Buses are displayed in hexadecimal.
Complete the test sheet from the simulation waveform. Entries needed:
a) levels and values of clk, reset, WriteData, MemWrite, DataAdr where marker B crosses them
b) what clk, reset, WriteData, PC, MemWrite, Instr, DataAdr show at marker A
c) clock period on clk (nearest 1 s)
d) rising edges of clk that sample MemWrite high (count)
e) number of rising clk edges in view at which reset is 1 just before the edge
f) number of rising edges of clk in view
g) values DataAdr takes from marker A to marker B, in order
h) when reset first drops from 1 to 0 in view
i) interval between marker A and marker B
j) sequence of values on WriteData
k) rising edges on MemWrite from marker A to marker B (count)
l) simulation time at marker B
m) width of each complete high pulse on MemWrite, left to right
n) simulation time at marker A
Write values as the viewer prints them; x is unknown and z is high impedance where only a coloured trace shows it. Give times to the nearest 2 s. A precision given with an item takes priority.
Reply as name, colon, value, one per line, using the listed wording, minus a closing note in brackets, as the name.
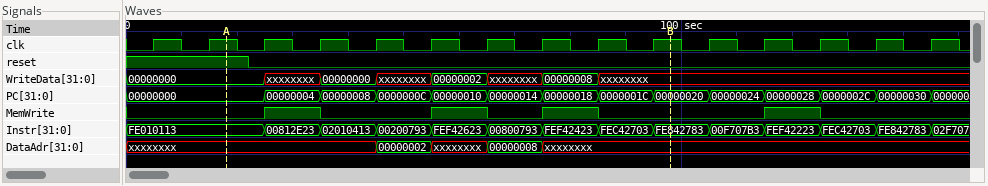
levels and values of clk, reset, WriteData, MemWrite, DataAdr where marker B crosses them: clk=1, reset=0, WriteData=xxxxxxxx, MemWrite=0, DataAdr=xxxxxxxx
what clk, reset, WriteData, PC, MemWrite, Instr, DataAdr show at marker A: clk=1, reset=1, WriteData=00000000, PC=00000000, MemWrite=0, Instr=FE010113, DataAdr=xxxxxxxx
clock period on clk: 10 s
rising edges of clk that sample MemWrite high: 4
number of rising clk edges in view at which reset is 1 just before the edge: 2
number of rising edges of clk in view: 15
values DataAdr takes from marker A to marker B, in order: xxxxxxxx, 00000002, xxxxxxxx, 00000008, xxxxxxxx
when reset first drops from 1 to 0 in view: 22 s
interval between marker A and marker B: 80 s
sequence of values on WriteData: 00000000, xxxxxxxx, 00000000, xxxxxxxx, 00000002, xxxxxxxx, 00000008, xxxxxxxx
rising edges on MemWrite from marker A to marker B: 3
simulation time at marker B: 98 s
width of each complete high pulse on MemWrite, left to right: 10 s, 10 s, 10 s, 10 s
simulation time at marker A: 18 s
